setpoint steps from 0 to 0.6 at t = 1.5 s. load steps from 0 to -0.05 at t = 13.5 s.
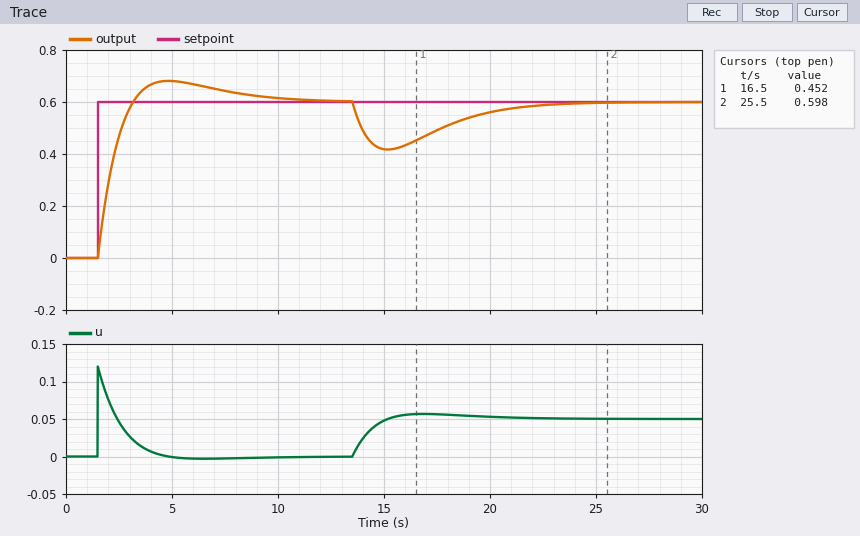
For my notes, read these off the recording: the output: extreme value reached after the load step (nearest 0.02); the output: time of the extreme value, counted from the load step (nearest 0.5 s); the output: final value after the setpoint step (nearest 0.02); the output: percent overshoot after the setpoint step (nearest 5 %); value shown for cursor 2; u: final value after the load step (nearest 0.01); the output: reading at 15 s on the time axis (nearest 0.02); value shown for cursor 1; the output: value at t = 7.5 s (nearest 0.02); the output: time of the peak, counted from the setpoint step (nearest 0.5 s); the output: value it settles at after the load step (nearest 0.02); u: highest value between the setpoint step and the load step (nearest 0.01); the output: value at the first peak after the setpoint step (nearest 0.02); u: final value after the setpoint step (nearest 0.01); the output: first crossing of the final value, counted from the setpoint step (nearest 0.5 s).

0.42
1.5 s
0.60
15 %
0.598
0.05
0.42
0.452
0.64
3.5 s
0.60
0.12
0.68
0.00
1.5 s
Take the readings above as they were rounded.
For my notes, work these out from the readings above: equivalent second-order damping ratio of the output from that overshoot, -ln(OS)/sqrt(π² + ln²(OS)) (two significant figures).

0.52
